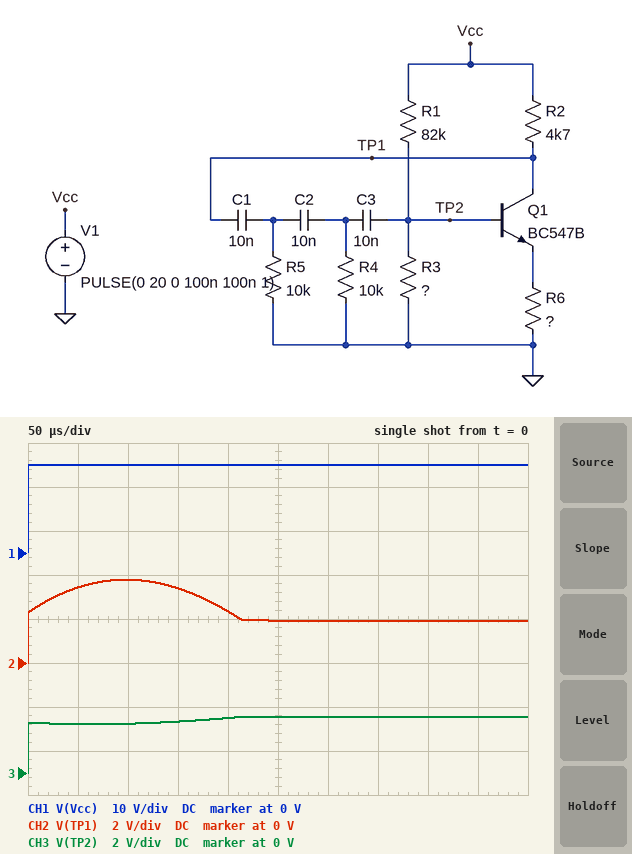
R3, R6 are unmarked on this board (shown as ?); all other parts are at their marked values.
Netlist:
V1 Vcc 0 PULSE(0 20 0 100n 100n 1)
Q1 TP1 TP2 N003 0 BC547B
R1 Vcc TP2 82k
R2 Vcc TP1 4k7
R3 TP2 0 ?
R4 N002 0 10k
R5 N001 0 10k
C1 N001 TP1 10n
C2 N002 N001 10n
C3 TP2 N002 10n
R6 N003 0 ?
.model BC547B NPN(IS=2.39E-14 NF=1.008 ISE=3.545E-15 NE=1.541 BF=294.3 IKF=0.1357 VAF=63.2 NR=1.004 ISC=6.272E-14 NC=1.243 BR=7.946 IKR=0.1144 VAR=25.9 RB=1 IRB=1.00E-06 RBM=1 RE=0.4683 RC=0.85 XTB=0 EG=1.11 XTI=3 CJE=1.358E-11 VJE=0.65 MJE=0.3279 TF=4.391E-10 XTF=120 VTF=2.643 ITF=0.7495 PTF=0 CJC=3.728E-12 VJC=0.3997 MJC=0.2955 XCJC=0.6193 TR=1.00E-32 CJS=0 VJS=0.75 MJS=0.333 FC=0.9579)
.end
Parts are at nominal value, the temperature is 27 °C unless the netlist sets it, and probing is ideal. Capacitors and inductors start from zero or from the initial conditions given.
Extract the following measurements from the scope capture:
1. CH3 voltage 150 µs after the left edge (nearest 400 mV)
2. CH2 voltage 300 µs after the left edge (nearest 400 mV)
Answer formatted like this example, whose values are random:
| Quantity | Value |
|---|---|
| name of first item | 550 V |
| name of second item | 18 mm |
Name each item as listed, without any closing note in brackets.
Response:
| Quantity | Value |
|---|---|
| CH3 voltage 150 µs after the left edge | 2.4 V |
| CH2 voltage 300 µs after the left edge | 2.0 V |
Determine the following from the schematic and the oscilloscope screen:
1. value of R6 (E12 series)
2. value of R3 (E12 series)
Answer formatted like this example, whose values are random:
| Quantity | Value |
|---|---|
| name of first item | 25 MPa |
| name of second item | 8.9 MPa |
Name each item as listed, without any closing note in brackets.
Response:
| Quantity | Value |
|---|---|
| value of R6 | 470 Ω |
| value of R3 | 27 kΩ |
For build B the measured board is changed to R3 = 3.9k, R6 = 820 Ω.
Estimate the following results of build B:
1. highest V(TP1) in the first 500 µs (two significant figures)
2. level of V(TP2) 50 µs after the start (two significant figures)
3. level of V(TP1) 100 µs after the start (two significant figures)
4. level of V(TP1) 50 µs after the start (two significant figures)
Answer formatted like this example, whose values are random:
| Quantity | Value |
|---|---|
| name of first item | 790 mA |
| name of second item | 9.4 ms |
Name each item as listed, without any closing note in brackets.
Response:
| Quantity | Value |
|---|---|
| highest V(TP1) in the first 500 µs | 19 V |
| level of V(TP2) 50 µs after the start | 1.4 V |
| level of V(TP1) 100 µs after the start | 16 V |
| level of V(TP1) 50 µs after the start | 11 V |
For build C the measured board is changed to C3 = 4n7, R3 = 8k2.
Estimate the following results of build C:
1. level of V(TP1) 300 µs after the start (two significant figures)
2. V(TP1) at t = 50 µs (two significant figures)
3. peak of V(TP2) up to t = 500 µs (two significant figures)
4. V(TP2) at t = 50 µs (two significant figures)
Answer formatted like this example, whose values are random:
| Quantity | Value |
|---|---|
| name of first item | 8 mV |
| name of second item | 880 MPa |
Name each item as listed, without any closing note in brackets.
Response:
| Quantity | Value |
|---|---|
| level of V(TP1) 300 µs after the start | 12 V |
| V(TP1) at t = 50 µs | 6.1 V |
| peak of V(TP2) up to t = 500 µs | 2.2 V |
| V(TP2) at t = 50 µs | 1.8 V |
